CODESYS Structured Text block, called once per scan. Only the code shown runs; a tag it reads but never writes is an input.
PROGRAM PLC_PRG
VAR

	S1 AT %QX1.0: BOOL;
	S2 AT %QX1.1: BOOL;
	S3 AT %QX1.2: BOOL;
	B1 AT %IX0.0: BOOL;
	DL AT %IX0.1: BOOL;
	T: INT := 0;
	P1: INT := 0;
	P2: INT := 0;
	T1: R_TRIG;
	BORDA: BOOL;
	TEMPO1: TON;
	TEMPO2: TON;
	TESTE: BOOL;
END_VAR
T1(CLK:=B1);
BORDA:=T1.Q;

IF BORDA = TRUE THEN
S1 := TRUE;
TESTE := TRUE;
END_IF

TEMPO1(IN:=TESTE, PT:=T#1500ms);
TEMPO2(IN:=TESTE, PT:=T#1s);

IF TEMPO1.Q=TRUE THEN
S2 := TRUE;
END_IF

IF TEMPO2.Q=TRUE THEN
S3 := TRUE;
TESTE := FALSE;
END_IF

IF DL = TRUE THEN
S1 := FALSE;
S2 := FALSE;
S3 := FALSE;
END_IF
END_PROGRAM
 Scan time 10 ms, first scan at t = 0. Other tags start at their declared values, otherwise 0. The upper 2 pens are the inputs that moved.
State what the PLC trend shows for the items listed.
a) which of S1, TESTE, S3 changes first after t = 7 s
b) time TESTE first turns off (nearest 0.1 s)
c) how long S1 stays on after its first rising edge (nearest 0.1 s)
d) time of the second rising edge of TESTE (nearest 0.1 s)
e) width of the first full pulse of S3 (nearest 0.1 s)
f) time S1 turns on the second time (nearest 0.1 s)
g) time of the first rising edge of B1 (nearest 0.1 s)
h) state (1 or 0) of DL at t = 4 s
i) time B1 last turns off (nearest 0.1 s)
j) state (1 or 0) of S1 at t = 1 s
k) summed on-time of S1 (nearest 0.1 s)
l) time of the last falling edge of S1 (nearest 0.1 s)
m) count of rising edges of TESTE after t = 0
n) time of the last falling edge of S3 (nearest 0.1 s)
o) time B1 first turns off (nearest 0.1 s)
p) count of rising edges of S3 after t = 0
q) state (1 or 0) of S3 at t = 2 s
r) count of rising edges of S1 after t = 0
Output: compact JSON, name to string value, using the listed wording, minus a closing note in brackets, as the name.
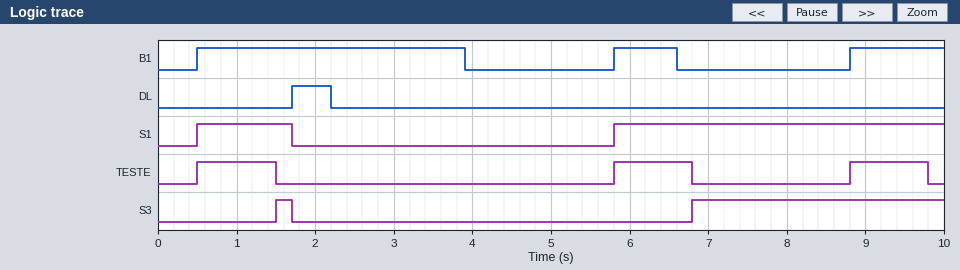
{"which of S1, TESTE, S3 changes first after t = 7 s": "TESTE", "time TESTE first turns off": "1.5 s", "how long S1 stays on after its first rising edge": "1.2 s", "time of the second rising edge of TESTE": "5.8 s", "width of the first full pulse of S3": "0.2 s", "time S1 turns on the second time": "5.8 s", "time of the first rising edge of B1": "0.5 s", "state (1 or 0) of DL at t = 4 s": "0", "time B1 last turns off": "6.6 s", "state (1 or 0) of S1 at t = 1 s": "1", "summed on-time of S1": "5.4 s", "time of the last falling edge of S1": "1.7 s", "count of rising edges of TESTE after t = 0": "3", "time of the last falling edge of S3": "1.7 s", "time B1 first turns off": "3.9 s", "count of rising edges of S3 after t = 0": "2", "state (1 or 0) of S3 at t = 2 s": "0", "count of rising edges of S1 after t = 0": "2"}
